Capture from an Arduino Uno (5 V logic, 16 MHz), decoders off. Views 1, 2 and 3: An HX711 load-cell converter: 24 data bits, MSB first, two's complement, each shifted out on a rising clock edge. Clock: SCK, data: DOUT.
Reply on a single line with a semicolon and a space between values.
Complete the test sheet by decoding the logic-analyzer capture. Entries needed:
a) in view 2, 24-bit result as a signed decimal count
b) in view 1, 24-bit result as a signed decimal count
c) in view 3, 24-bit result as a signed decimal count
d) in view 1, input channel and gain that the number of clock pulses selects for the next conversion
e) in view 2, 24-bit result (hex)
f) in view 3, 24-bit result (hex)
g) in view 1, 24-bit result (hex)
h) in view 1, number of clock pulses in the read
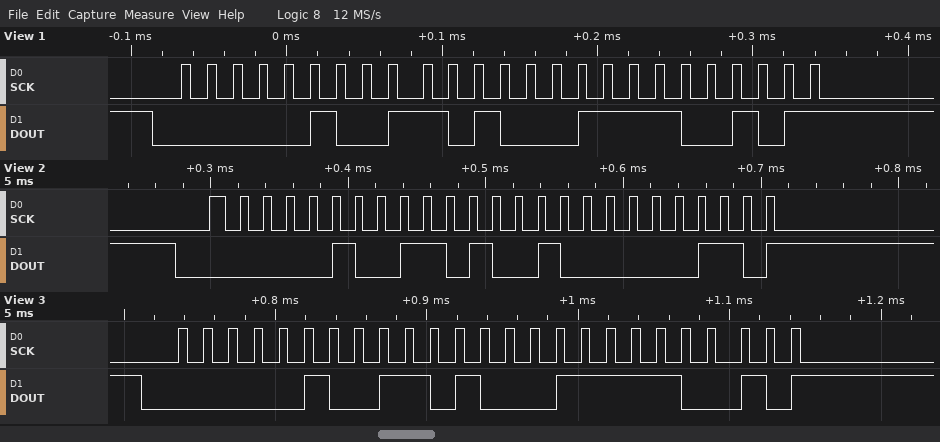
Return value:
315910; 315877; 315890; channel A, gain 128; 0x04D206; 0x04D1F2; 0x04D1E5; 25
